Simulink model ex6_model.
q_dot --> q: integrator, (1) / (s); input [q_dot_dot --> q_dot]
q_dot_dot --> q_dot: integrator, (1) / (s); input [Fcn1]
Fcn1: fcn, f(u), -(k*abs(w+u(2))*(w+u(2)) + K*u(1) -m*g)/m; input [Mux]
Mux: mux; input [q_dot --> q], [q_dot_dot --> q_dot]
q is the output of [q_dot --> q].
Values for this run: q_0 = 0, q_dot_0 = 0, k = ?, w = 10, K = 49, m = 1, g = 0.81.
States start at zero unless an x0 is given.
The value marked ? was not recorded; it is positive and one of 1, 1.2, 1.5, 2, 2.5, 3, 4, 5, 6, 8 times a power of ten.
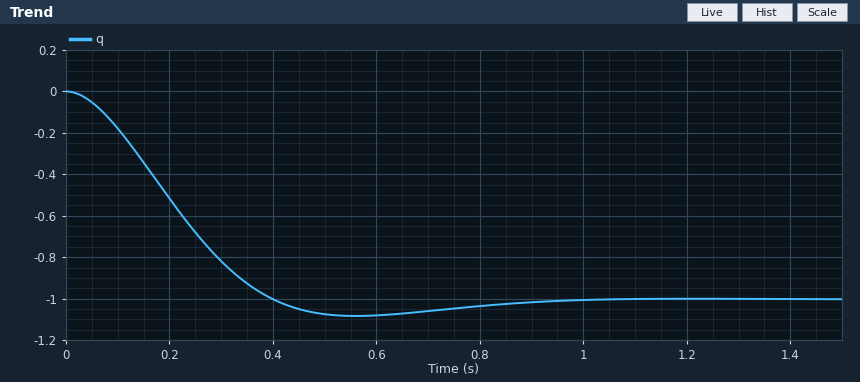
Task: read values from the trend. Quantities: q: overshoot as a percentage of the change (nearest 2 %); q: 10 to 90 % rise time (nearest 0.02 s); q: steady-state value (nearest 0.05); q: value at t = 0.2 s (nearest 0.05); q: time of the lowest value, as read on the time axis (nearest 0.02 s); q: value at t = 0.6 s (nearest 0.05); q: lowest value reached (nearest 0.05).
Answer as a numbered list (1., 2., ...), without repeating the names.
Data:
1. 8 %
2. 0.26 s
3. -1.00
4. -0.50
5. 0.56 s
6. -1.10
7. -1.10
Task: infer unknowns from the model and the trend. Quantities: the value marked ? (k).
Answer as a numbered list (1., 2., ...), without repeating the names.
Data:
1. 0.5
